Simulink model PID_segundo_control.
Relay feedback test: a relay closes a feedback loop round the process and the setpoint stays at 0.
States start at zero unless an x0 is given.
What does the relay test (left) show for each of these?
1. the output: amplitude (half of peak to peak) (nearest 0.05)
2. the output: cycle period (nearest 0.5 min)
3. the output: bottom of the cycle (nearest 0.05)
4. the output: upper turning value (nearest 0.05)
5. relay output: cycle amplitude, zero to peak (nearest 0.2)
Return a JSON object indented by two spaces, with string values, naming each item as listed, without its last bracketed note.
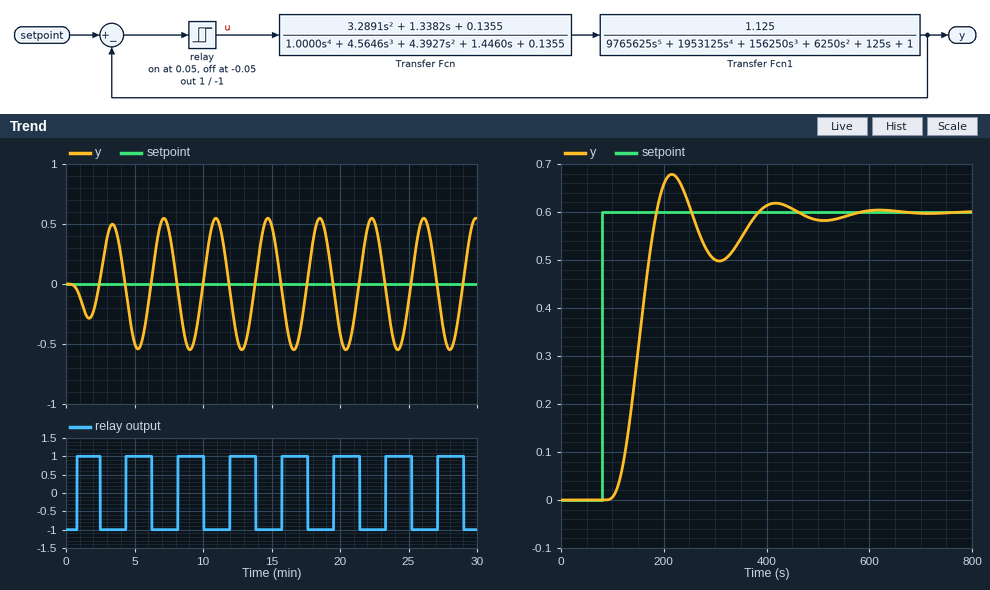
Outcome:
{
  "the output: amplitude (half of peak to peak)": "0.55",
  "the output: cycle period": "4.0 min",
  "the output: bottom of the cycle": "-0.55",
  "the output: upper turning value": "0.55",
  "relay output: cycle amplitude, zero to peak": "1.0"
}
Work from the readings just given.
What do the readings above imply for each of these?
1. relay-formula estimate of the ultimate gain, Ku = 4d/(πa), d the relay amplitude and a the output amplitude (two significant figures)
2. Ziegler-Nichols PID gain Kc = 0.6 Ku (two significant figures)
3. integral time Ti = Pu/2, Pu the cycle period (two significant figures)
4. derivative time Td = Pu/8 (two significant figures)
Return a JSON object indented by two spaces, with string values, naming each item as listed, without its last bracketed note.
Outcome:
{
  "relay-formula estimate of the ultimate gain, Ku = 4d/(πa), d the relay amplitude and a the output amplitude": "2.3",
  "Ziegler-Nichols PID gain Kc = 0.6 Ku": "1.4",
  "integral time Ti = Pu/2, Pu the cycle period": "2.0 min",
  "derivative time Td = Pu/8": "0.50 min"
}
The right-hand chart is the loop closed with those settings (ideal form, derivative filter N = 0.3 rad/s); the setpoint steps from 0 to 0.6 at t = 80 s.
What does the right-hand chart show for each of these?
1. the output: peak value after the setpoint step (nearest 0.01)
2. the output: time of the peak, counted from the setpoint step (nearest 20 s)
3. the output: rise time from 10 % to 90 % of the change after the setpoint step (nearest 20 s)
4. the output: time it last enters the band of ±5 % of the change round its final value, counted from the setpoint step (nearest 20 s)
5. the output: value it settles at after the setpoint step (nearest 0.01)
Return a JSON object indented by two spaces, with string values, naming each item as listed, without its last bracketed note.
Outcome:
{
  "the output: peak value after the setpoint step": "0.68",
  "the output: time of the peak, counted from the setpoint step": "140 s",
  "the output: rise time from 10 % to 90 % of the change after the setpoint step": "60 s",
  "the output: time it last enters the band of ±5 % of the change round its final value, counted from the setpoint step": "280 s",
  "the output: value it settles at after the setpoint step": "0.60"
}
